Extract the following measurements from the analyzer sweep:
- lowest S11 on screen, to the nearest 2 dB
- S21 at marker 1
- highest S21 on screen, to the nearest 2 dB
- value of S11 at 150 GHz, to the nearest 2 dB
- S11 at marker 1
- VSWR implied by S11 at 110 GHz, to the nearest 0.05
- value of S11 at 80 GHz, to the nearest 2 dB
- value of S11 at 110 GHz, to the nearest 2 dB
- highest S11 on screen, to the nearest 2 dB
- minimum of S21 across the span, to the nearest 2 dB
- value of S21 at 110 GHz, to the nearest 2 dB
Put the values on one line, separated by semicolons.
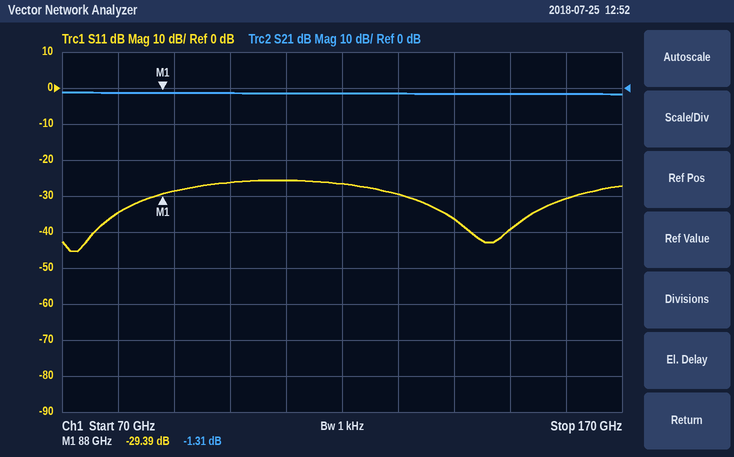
-46 dB; -1.31 dB; -2 dB; -40 dB; -29.39 dB; 1.10; -34 dB; -26 dB; -26 dB; -2 dB; -2 dB
